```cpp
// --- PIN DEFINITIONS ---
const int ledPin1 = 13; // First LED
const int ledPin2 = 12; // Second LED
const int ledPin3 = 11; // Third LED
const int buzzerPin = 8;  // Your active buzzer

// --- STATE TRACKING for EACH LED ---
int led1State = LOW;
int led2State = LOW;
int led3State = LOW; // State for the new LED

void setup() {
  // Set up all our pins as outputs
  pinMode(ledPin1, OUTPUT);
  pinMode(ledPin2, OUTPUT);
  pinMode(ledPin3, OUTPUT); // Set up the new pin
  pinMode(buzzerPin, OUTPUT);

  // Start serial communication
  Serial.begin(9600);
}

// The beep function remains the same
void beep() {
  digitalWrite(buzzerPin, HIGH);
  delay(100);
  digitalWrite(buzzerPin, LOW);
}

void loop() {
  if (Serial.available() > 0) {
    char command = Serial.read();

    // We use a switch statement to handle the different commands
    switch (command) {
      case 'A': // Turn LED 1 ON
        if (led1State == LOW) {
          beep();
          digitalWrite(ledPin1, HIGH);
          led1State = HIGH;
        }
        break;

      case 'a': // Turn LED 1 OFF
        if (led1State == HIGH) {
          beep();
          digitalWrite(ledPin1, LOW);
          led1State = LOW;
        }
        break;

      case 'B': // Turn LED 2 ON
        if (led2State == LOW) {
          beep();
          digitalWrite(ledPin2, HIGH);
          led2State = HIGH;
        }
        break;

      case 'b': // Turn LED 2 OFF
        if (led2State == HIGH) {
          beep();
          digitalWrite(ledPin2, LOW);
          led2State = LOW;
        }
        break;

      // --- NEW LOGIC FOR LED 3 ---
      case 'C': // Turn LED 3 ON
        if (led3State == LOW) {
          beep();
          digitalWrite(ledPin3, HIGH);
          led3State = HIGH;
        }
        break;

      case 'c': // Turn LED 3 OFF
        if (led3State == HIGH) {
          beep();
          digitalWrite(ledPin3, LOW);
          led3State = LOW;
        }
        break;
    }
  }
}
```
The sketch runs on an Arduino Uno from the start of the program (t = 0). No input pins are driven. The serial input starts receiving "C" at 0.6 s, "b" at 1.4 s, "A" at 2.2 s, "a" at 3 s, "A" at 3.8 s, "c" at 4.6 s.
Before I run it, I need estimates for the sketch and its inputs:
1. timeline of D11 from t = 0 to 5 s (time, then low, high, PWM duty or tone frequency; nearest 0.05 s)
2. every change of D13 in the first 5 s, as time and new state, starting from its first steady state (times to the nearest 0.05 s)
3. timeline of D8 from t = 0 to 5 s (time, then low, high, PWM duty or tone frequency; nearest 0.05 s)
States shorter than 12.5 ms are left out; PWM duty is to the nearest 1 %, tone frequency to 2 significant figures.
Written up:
0 s low; 0.7 s high; 4.7 s low
0 s low; 2.3 s high; 3.1 s low; 3.9 s high
0 s low; 0.6 s high; 0.7 s low; 2.2 s high; 2.3 s low; 3 s high; 3.1 s low; 3.8 s high; 3.9 s low; 4.6 s high; 4.7 s low
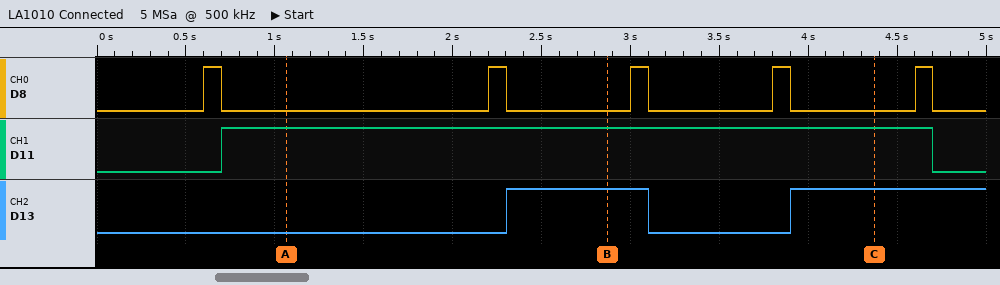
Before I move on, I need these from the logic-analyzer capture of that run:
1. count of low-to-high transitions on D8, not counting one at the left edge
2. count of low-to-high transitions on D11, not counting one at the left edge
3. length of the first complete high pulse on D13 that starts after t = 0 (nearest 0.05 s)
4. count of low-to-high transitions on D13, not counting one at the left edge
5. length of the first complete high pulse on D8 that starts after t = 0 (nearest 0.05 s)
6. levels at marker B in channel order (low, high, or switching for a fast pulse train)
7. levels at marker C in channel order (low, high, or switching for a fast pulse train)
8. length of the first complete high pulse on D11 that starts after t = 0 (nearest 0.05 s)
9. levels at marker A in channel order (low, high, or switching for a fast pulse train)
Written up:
5
1
0.80 s
2
0.10 s
D8 low, D11 high, D13 high
D8 low, D11 high, D13 high
4.00 s
D8 low, D11 high, D13 low
